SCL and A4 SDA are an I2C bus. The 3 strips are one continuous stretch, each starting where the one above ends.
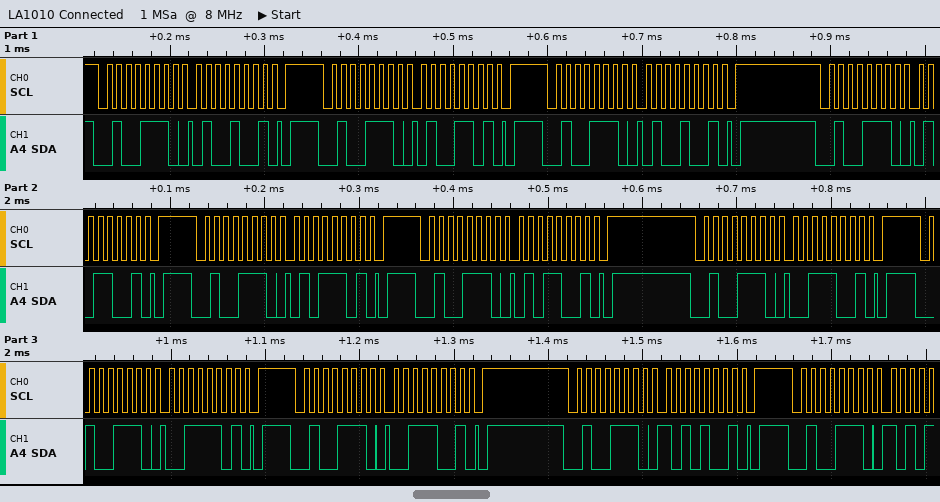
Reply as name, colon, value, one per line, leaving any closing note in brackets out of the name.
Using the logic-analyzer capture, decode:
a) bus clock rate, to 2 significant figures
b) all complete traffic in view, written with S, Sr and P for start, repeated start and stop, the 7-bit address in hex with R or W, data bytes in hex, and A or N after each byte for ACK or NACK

bus clock rate, to 2 significant figures: 100 kHz
all complete traffic in view, written with S, Sr and P for start, repeated start and stop, the 7-bit address in hex with R or W, data bytes in hex, and A or N after each byte for ACK or NACK: S 27W A 49 A P S 27W A 4D A P S 27W A 49 A P S 27W A 59 A P S 27W A 5D A P S 27W A 59 A P S 27W A 39 A P S 27W A 3D A P S 27W A 39 A P S 27W A A9 A P S 27W A
